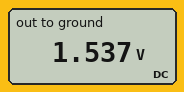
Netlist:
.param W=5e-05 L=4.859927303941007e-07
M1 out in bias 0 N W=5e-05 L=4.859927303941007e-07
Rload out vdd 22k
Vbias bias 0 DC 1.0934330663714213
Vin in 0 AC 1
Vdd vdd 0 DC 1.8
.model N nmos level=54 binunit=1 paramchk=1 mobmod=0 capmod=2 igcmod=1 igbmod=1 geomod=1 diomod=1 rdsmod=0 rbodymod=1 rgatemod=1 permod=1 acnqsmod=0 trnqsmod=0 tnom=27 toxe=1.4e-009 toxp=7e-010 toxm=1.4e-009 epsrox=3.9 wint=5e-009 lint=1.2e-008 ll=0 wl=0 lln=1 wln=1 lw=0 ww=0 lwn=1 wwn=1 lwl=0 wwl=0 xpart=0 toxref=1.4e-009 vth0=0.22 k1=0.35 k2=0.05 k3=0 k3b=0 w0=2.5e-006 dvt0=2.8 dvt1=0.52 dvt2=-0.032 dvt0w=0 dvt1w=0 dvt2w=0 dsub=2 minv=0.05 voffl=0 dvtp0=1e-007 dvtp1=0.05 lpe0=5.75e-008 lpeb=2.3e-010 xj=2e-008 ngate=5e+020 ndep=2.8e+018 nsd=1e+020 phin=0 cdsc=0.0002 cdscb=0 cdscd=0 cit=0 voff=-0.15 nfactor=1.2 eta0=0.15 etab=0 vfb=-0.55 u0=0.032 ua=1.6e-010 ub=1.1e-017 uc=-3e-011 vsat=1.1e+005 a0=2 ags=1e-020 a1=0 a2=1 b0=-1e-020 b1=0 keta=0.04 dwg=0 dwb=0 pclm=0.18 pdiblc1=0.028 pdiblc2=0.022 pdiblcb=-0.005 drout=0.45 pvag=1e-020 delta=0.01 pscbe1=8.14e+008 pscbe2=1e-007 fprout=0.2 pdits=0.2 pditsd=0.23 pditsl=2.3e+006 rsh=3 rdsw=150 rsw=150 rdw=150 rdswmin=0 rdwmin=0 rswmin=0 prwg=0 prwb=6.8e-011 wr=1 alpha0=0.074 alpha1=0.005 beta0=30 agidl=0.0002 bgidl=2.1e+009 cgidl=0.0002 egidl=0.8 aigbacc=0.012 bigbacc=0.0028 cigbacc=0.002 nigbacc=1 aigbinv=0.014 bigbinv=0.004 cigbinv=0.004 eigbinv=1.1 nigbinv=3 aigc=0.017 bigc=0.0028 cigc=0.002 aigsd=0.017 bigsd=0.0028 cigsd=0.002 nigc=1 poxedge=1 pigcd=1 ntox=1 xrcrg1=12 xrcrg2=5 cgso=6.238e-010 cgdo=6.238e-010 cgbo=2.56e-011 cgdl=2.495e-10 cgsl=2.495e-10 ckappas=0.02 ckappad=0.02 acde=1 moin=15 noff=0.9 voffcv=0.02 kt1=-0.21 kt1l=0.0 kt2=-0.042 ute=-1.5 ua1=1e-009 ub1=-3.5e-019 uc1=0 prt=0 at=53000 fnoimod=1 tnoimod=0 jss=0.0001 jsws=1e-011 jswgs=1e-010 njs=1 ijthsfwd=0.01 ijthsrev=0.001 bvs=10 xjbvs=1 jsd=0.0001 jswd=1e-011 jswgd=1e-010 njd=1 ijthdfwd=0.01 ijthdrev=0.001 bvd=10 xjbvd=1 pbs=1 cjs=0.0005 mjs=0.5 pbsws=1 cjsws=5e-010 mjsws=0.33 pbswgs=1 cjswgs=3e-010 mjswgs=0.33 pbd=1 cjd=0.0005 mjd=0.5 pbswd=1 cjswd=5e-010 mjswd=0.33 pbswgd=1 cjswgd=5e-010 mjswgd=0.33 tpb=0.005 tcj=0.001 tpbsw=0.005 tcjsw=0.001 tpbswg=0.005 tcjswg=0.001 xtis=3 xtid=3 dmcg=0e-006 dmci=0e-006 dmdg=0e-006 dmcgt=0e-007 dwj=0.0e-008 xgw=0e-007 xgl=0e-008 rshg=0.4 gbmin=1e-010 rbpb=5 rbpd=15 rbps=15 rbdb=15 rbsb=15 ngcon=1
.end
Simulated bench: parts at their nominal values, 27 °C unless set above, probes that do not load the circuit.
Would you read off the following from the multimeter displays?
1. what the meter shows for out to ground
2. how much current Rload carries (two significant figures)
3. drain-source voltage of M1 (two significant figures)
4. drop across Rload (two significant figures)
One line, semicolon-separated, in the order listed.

1.537 V; 12 µA; 440 mV; 260 mV
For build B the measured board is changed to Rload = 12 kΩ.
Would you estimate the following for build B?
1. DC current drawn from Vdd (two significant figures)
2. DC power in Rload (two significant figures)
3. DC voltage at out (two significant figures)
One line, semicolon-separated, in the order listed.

19 µA; 4.5 µW; 1.6 V
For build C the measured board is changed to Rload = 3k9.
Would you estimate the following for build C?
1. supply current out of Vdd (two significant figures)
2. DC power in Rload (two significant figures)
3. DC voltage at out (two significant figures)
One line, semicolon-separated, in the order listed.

45 µA; 7.9 µW; 1.6 V
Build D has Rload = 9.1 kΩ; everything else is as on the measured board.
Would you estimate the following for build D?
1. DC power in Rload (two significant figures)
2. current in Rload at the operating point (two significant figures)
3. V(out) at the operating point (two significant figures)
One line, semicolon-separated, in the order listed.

5.3 µW; 24 µA; 1.6 V
